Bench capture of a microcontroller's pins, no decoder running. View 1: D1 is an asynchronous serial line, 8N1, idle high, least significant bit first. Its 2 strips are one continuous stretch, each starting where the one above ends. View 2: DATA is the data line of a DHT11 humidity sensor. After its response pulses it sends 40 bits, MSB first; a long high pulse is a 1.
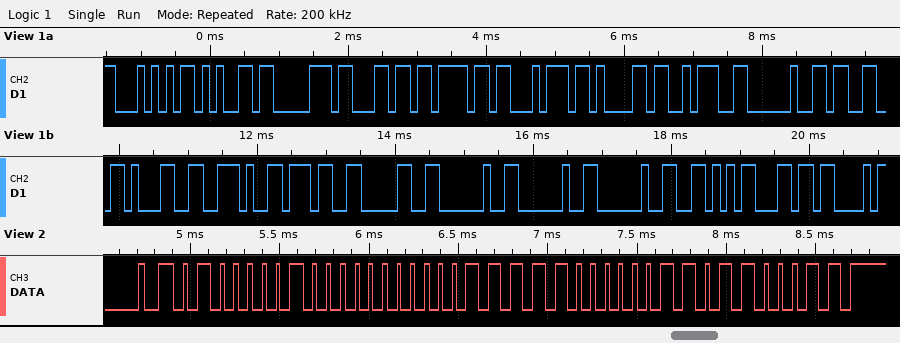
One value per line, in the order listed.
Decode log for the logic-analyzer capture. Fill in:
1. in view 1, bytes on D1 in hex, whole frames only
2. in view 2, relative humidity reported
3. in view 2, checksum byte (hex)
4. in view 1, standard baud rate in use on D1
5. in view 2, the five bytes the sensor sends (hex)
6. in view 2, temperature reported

54 65 70 6C 6F 74 61 3A 20 33 31 2E 37 30 20 20 20 56 6C
65 %
0x63
9600 baud
41 00 1F 03 63
31.3 °C
